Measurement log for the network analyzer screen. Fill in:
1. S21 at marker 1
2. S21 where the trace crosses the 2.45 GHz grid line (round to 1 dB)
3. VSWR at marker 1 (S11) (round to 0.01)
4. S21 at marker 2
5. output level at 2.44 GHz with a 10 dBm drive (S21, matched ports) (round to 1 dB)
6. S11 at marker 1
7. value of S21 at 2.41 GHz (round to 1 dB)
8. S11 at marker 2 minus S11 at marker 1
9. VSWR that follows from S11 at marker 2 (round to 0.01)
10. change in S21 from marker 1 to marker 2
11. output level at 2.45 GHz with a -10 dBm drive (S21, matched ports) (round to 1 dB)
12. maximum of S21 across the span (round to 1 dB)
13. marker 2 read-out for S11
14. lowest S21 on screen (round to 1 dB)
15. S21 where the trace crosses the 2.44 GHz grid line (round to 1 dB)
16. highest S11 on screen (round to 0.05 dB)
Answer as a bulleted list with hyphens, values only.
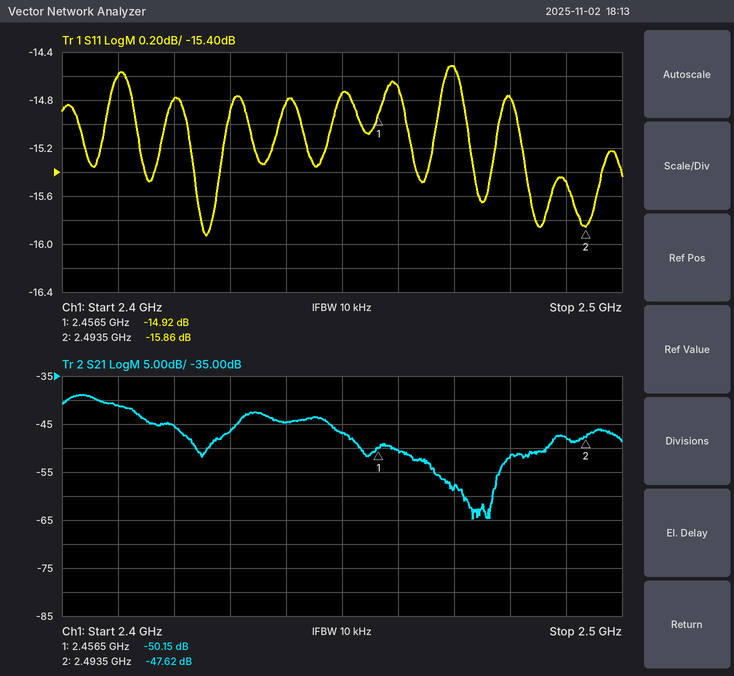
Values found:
- -50.15 dB
- -47 dB
- 1.44
- -47.62 dB
- -35 dBm
- -14.92 dB
- -41 dB
- -0.94 dB
- 1.38
- 2.53 dB
- -57 dBm
- -39 dB
- -15.86 dB
- -65 dB
- -45 dB
- -14.50 dB
